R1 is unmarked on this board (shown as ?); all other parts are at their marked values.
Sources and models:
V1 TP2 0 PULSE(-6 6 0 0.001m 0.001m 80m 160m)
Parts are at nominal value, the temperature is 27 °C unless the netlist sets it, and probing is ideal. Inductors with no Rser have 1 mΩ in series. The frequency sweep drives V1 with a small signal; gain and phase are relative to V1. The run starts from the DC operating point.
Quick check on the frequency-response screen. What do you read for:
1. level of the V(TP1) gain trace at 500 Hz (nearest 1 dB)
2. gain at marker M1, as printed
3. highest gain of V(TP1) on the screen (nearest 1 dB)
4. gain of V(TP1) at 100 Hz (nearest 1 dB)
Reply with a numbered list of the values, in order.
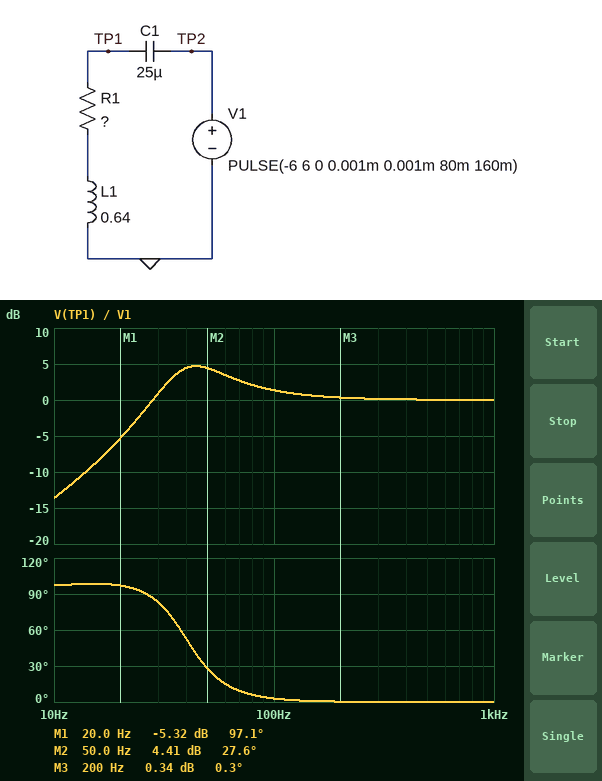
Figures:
1. 0 dB
2. -5.32 dB
3. 5 dB
4. 1 dB
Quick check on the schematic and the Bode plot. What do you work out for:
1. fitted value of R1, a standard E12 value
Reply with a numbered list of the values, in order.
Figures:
1. 120 Ω
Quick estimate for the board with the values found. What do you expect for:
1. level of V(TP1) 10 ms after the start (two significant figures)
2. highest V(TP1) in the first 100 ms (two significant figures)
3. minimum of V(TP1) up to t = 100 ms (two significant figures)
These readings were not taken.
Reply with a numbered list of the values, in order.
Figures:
1. -1.8 V
2. 12 V
3. -12 V
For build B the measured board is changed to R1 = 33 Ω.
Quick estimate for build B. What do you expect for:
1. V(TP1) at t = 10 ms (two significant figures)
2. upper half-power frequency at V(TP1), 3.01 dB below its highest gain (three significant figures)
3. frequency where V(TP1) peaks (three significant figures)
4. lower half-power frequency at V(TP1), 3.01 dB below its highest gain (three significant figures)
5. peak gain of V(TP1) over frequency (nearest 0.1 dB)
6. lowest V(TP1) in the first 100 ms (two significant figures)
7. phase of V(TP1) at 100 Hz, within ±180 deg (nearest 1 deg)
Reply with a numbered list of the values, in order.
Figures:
1. -6.8 V
2. 45.2 Hz
3. 40.2 Hz
4. 36.5 Hz
5. 13.9 dB
6. -11 V
7. 1 deg
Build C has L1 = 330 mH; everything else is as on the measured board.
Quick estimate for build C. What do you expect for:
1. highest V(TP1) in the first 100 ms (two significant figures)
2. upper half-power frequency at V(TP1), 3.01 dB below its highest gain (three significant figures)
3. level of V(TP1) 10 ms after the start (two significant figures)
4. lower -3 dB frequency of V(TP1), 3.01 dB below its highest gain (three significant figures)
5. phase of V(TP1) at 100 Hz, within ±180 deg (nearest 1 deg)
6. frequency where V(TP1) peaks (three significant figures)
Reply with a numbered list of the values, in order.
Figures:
1. 12 V
2. 430 Hz
3. -1.7 V
4. 39.7 Hz
5. 10 deg
6. 65.4 Hz
